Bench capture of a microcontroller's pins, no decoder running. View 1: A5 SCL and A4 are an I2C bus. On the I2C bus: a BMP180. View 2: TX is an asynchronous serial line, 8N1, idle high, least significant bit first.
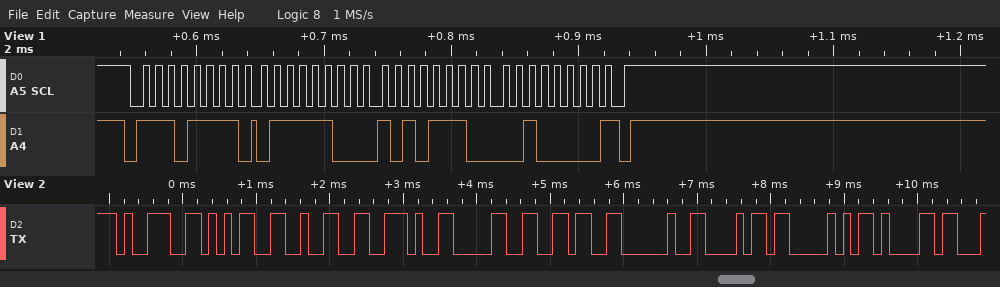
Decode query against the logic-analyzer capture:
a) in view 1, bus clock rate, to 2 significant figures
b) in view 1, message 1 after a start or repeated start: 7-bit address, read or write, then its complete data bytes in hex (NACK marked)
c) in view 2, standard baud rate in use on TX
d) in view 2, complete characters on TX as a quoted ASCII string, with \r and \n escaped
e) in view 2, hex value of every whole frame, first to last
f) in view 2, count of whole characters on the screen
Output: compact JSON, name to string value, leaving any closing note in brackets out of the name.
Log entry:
{"in view 1, bus clock rate, to 2 significant figures": "100 kHz", "in view 1, message 1 after a start or repeated start: 7-bit address, read or write, then its complete data bytes in hex": "0x77 read: 7C AE 20 NACK", "in view 2, standard baud rate in use on TX": "9600 baud", "in view 2, complete characters on TX as a quoted ASCII string, with \\r and \\n escaped": "\"952.06 hPa\"", "in view 2, hex value of every whole frame, first to last": "39 35 32 2E 30 36 20 68 50 61", "in view 2, count of whole characters on the screen": "10"}
